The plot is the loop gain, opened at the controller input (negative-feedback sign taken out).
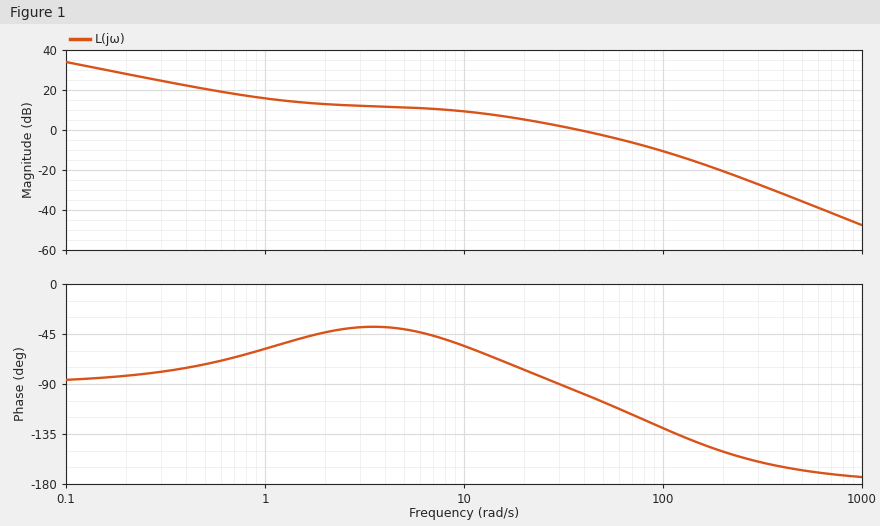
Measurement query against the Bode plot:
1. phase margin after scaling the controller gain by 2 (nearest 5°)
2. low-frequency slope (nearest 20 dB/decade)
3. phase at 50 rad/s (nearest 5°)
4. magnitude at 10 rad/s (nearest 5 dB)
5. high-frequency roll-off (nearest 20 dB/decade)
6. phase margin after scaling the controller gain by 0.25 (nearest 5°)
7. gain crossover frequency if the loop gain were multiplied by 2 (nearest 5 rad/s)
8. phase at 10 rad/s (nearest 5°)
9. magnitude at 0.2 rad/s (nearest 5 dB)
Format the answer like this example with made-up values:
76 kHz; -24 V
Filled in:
65°; -20 dB/decade; -105°; 10 dB; -40 dB/decade; 140°; 70 rad/s; -55°; 30 dB
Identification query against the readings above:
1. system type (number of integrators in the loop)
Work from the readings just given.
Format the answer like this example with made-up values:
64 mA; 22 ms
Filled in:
1
